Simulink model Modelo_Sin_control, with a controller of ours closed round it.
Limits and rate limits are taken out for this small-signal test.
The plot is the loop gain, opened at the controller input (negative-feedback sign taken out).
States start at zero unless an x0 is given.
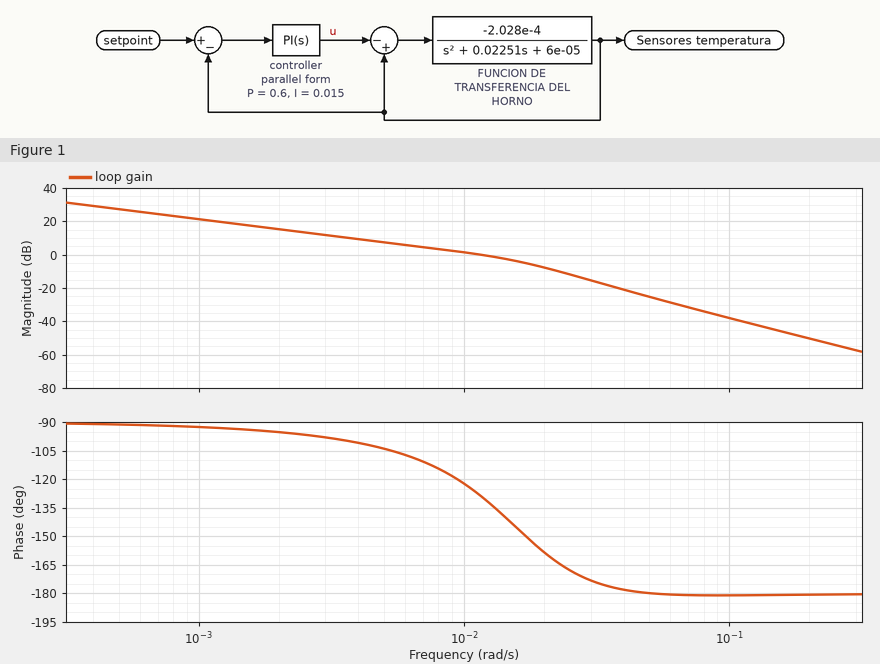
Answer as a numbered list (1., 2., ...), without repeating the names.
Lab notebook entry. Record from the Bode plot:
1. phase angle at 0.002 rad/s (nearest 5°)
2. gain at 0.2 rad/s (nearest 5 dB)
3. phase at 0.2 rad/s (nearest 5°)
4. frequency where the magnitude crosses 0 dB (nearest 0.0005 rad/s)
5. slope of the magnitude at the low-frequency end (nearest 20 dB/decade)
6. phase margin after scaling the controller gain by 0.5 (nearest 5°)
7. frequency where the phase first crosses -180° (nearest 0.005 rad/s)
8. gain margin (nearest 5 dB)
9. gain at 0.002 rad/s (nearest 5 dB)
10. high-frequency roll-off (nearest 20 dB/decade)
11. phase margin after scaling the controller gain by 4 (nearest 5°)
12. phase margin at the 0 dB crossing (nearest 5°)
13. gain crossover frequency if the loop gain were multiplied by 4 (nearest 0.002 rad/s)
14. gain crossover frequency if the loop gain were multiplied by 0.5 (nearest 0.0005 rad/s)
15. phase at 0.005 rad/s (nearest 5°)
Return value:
1. -95°
2. -50 dB
3. -180°
4. 0.0115 rad/s
5. -20 dB/decade
6. 75°
7. 0.050 rad/s
8. 25 dB
9. 15 dB
10. -40 dB/decade
11. 10°
12. 50°
13. 0.026 rad/s
14. 0.0060 rad/s
15. -105°
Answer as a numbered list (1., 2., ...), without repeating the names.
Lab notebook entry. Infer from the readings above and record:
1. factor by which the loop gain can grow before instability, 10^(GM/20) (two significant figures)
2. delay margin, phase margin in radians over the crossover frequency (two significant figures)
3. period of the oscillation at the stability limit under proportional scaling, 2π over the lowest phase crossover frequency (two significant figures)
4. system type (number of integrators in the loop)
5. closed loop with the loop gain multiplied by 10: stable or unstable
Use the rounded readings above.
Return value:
1. 18
2. 76 s
3. 130 s
4. 1
5. stable
